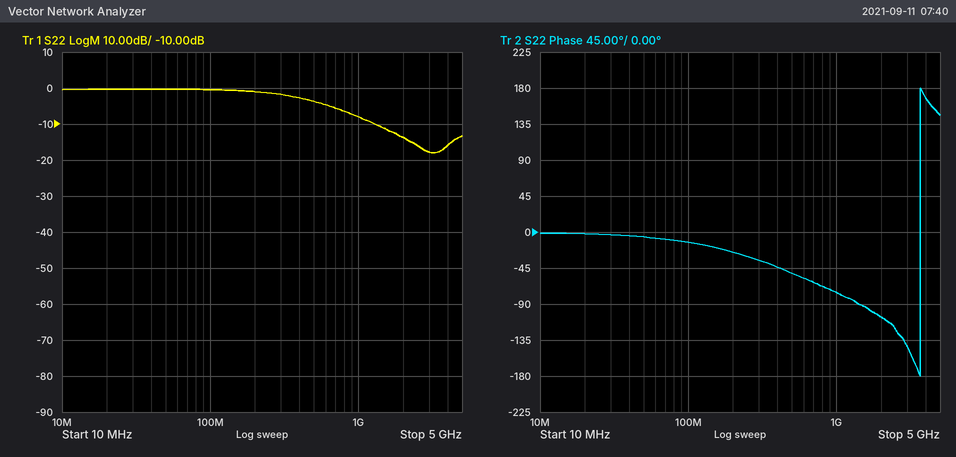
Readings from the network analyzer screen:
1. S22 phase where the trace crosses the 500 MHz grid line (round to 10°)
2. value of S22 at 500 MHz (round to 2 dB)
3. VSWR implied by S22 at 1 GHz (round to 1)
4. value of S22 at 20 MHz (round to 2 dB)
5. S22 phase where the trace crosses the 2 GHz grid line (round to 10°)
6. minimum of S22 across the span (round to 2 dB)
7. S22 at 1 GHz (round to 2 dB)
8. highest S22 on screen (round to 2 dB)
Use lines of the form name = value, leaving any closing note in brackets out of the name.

S22 phase where the trace crosses the 500 MHz grid line = -50°
value of S22 at 500 MHz = -4 dB
VSWR implied by S22 at 1 GHz = 2
value of S22 at 20 MHz = 0 dB
S22 phase where the trace crosses the 2 GHz grid line = -110°
minimum of S22 across the span = -18 dB
S22 at 1 GHz = -8 dB
highest S22 on screen = 0 dB
